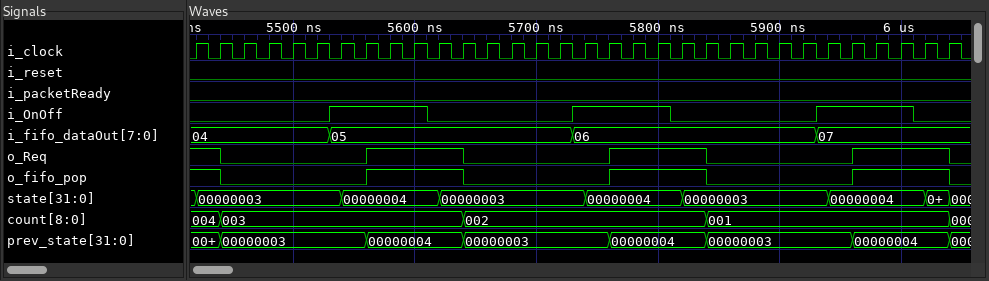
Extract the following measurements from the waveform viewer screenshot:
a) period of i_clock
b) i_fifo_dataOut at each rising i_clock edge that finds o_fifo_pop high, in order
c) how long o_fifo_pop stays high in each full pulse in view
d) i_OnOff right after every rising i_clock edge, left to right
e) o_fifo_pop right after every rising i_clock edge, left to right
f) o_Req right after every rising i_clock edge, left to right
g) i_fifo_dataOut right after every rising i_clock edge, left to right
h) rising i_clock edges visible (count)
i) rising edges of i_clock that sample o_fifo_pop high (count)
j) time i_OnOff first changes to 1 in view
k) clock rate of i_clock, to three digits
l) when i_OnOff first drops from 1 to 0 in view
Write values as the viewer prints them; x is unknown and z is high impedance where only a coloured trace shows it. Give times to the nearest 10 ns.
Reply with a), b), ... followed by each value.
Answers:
a) 20 ns
b) 04, 04, 05, 05, 05, 05, 06, 06, 06, 06, 07, 07, 07, 07
c) 80 ns, 80 ns, 80 ns
d) 0 0 0 0 0 0 1 1 1 1 0 0 0 0 0 0 1 1 1 1 0 0 0 0 0 0 1 1 1 1 0 0
e) 1 0 0 0 0 0 0 1 1 1 1 0 0 0 0 0 0 1 1 1 1 0 0 0 0 0 0 1 1 1 1 0
f) 1 0 0 0 0 0 0 1 1 1 1 0 0 0 0 0 0 1 1 1 1 0 0 0 0 0 0 1 1 1 1 0
g) 04, 04, 04, 04, 04, 04, 05, 05, 05, 05, 05, 05, 05, 05, 05, 05, 06, 06, 06, 06, 06, 06, 06, 06, 06, 06, 07, 07, 07, 07, 07, 07
h) 32
i) 14
j) 5530 ns
k) 50.0 MHz
l) 5610 ns
